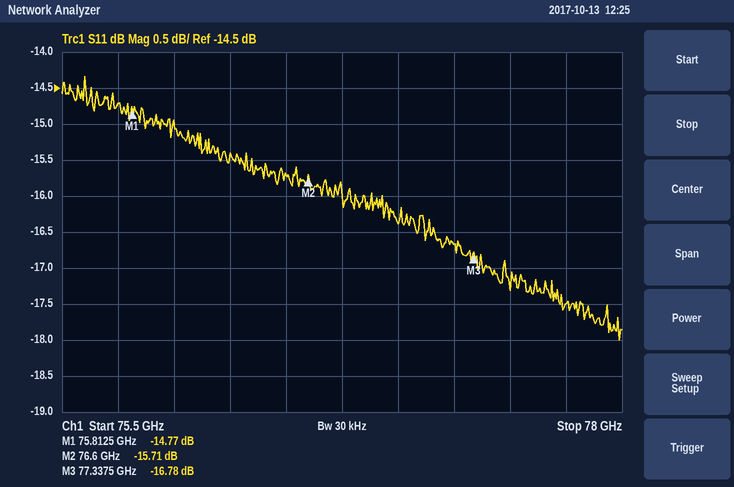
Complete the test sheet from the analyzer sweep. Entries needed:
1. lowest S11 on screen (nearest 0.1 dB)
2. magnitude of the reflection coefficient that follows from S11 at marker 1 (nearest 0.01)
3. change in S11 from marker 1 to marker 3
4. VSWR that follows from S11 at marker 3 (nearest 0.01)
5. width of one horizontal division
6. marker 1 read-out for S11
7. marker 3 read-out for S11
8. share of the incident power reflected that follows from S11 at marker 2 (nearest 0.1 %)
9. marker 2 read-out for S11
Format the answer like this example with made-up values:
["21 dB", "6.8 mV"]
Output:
["-18.0 dB", "0.18", "-2.01 dB", "1.34", "250 MHz", "-14.77 dB", "-16.78 dB", "2.7 %", "-15.71 dB"]
